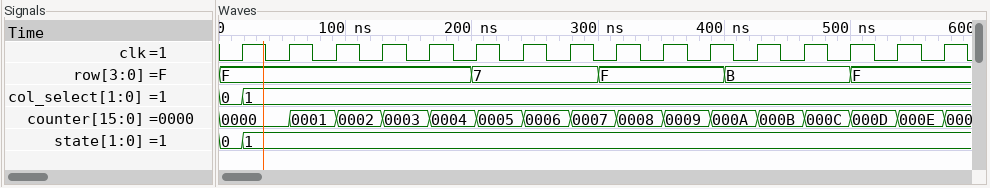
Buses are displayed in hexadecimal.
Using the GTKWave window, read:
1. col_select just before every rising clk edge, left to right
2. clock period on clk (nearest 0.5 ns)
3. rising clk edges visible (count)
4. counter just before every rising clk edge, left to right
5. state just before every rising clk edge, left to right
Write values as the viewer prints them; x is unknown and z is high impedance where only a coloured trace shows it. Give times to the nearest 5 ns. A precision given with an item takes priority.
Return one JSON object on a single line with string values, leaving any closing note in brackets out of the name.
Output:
{"col_select just before every rising clk edge, left to right": "0, 1, 1, 1, 1, 1, 1, 1, 1, 1, 1, 1, 1, 1, 1, 1", "clock period on clk": "37 ns", "rising clk edges visible": "16", "counter just before every rising clk edge, left to right": "0000, 0000, 0001, 0002, 0003, 0004, 0005, 0006, 0007, 0008, 0009, 000A, 000B, 000C, 000D, 000E", "state just before every rising clk edge, left to right": "0, 1, 1, 1, 1, 1, 1, 1, 1, 1, 1, 1, 1, 1, 1, 1"}
